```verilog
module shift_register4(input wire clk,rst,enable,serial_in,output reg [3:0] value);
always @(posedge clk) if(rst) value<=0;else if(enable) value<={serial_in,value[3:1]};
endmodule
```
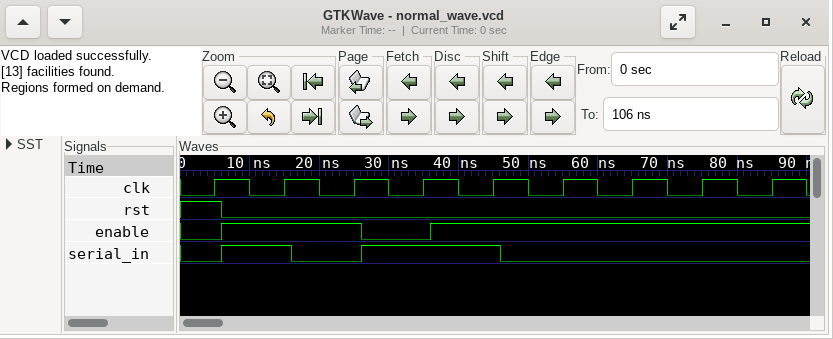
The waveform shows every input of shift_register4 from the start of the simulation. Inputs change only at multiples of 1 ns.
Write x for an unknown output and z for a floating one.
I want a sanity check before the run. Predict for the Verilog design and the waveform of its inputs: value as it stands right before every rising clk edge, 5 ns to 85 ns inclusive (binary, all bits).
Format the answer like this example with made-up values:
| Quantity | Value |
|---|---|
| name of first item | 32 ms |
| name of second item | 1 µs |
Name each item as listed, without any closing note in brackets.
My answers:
| Quantity | Value |
|---|---|
| value as it stands right before every rising clk edge, 5 ns to 85 ns inclusive | x, 0000, 1000, 0100, 0100, 1010, 0101, 0010, 0001 |
